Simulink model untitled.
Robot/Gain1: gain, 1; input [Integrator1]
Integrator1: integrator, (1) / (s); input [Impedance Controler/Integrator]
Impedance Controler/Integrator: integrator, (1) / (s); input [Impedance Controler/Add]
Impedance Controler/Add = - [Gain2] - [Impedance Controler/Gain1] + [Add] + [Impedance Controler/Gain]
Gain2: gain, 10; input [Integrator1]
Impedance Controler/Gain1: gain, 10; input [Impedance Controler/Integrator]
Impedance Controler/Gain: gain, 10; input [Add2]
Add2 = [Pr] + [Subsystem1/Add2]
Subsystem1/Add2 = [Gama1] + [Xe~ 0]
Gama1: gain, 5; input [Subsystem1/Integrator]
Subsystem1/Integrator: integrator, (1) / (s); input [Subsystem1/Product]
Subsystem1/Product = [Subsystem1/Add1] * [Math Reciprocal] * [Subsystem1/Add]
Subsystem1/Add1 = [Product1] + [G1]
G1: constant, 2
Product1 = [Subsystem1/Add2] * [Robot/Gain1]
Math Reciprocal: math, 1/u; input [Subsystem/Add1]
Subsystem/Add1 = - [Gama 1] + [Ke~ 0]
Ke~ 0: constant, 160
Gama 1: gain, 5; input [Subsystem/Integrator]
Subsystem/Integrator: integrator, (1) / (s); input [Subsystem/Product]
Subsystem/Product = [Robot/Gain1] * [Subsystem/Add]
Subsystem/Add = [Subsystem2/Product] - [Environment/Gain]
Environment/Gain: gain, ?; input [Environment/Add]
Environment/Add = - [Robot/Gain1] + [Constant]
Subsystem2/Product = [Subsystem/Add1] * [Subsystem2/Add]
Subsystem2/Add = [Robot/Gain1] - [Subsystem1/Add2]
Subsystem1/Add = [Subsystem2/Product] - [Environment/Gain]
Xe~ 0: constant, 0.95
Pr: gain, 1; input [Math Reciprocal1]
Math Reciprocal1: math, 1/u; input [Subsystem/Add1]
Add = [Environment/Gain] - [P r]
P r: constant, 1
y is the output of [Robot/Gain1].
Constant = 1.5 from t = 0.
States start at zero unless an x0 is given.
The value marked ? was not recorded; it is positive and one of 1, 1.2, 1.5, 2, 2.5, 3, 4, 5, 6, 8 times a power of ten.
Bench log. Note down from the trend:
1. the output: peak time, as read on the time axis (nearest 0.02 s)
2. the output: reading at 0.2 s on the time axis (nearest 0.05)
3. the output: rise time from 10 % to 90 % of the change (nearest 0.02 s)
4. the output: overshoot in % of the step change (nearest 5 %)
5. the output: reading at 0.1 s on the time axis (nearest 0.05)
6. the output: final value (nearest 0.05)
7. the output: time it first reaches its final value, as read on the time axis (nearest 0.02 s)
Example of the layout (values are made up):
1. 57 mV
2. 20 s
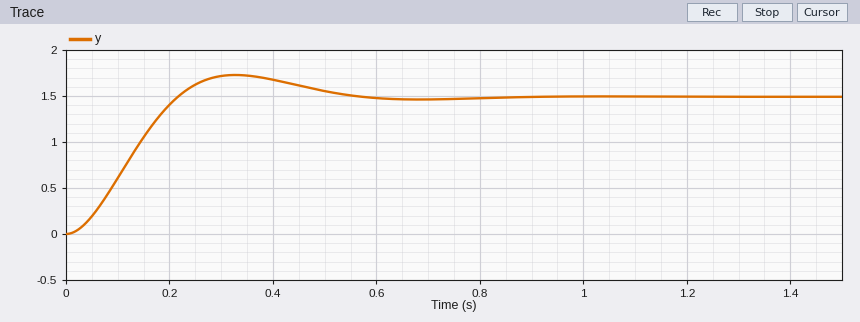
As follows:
1. 0.32 s
2. 1.40
3. 0.14 s
4. 15 %
5. 0.60
6. 1.50
7. 0.22 s
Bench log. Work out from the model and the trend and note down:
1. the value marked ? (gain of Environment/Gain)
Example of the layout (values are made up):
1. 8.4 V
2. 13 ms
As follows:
1. 120
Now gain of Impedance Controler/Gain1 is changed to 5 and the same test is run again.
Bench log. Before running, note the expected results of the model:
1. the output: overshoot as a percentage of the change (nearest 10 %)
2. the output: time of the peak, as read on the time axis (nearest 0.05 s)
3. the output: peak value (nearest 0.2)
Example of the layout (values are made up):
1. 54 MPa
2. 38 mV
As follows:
1. 40 %
2. 0.30 s
3. 2.2
